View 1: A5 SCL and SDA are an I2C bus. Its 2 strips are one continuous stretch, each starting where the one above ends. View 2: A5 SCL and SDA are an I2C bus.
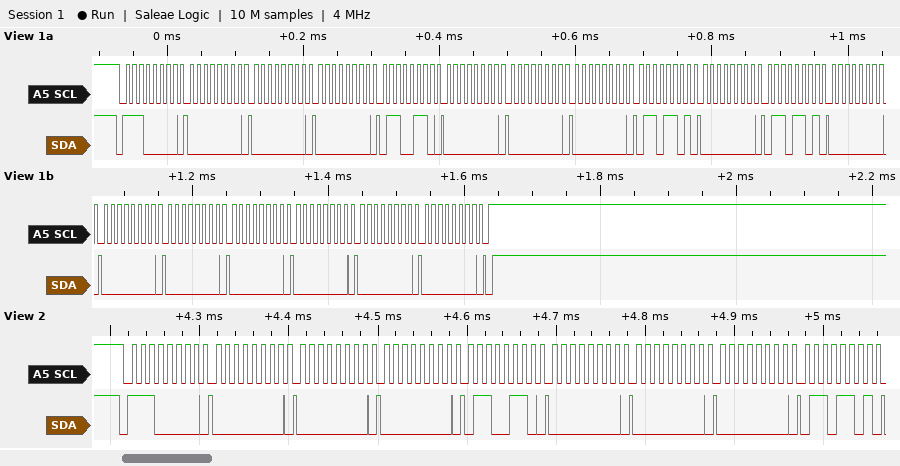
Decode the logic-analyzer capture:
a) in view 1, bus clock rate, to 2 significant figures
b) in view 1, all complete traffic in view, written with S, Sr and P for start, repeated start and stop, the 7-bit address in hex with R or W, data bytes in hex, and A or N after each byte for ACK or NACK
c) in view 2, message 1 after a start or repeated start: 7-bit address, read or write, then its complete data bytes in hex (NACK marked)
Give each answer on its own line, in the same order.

100 kHz
S 70W A 00 A 00 A 00 A 66 A 00 A 00 A 00 A 6D A 00 A 6D A 00 A 00 A 00 A 00 A 00 A 00 A 00 A P
0x70 write: 00 00 00 66 00 00 00 6D
